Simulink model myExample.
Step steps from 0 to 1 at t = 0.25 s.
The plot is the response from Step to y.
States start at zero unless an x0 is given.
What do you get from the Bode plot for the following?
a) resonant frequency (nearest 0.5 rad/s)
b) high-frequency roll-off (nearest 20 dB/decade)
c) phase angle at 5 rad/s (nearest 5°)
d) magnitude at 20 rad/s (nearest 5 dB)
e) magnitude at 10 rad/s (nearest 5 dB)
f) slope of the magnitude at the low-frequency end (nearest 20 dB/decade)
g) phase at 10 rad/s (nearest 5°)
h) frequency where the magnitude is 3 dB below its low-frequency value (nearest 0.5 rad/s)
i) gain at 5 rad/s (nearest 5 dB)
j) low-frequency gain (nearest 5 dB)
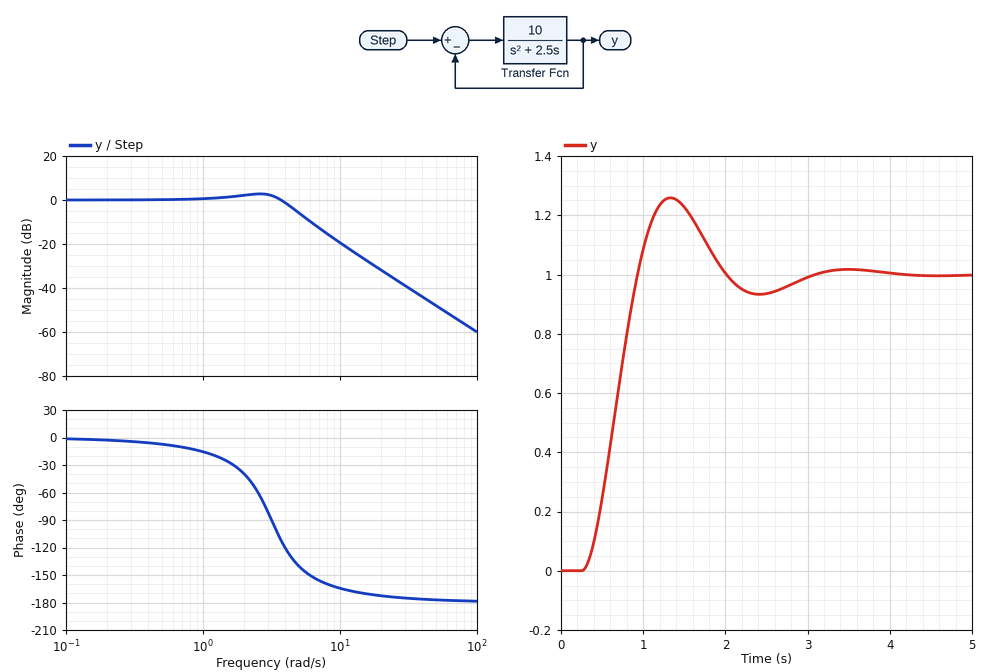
2.5 rad/s
-40 dB/decade
-140°
-30 dB
-20 dB
0 dB/decade
-165°
4.5 rad/s
-5 dB
0 dB
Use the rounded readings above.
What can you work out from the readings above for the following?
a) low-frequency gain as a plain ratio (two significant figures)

1.0
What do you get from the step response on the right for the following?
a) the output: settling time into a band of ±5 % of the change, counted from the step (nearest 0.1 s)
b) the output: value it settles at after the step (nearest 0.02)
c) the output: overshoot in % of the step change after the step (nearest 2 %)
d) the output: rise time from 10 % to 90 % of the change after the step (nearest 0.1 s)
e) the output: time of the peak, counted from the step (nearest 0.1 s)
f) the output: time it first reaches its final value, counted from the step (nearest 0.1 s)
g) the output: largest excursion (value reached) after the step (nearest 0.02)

2.4 s
1.00
26 %
0.5 s
1.1 s
0.7 s
1.26
